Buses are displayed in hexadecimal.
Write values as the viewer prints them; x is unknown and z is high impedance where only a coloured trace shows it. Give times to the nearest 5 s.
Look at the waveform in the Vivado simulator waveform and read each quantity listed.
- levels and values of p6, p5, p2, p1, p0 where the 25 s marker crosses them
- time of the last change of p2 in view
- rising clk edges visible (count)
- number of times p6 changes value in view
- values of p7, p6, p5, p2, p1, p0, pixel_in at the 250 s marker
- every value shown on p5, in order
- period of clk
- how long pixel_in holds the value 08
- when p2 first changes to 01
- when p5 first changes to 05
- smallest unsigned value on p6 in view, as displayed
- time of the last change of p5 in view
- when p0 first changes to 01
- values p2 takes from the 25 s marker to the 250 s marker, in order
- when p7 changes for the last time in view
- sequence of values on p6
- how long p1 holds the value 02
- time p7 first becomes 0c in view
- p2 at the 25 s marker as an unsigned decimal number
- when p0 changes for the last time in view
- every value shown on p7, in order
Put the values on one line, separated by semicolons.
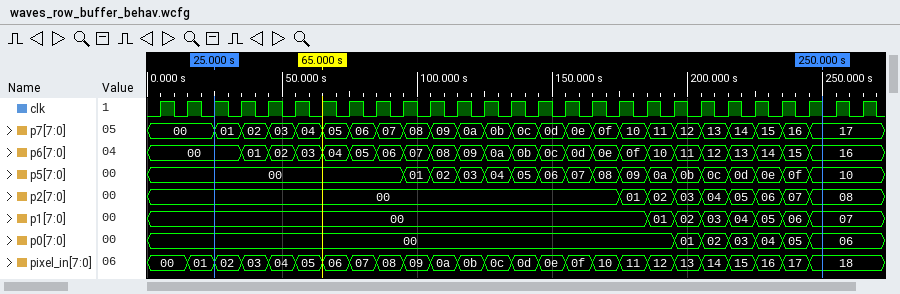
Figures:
p6=00, p5=00, p2=00, p1=00, p0=00; 245 s; 27; 22; p7=17, p6=16, p5=10, p2=08, p1=07, p0=06, pixel_in=18; 00, 01, 02, 03, 04, 05, 06, 07, 08, 09, 0a, 0b, 0c, 0d, 0e, 0f, 10; 10 s; 10 s; 175 s; 135 s; 00; 245 s; 195 s; 00, 01, 02, 03, 04, 05, 06, 07, 08; 245 s; 00, 01, 02, 03, 04, 05, 06, 07, 08, 09, 0a, 0b, 0c, 0d, 0e, 0f, 10, 11, 12, 13, 14, 15, 16; 10 s; 135 s; 0; 245 s; 00, 01, 02, 03, 04, 05, 06, 07, 08, 09, 0a, 0b, 0c, 0d, 0e, 0f, 10, 11, 12, 13, 14, 15, 16, 17
